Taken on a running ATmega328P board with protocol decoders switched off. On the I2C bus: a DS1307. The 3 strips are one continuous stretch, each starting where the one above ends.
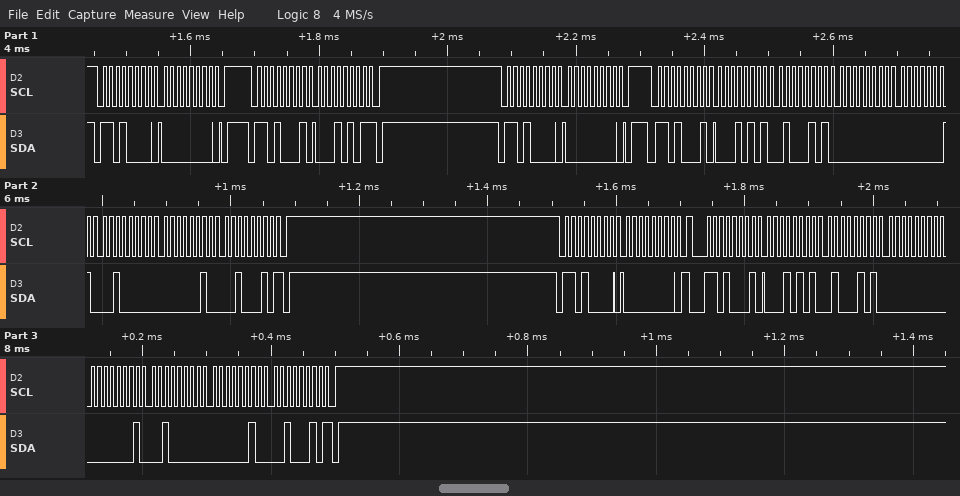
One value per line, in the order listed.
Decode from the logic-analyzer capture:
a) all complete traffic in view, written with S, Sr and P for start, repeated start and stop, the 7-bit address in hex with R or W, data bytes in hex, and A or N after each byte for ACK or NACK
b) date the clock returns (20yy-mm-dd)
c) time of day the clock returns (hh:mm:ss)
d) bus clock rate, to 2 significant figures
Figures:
S 68W A 00 A P S 68R A 15 N P S 68W A 00 A P S 68R A 15 A 45 A 00 A 01 A 20 A 02 A 22 N P S 68W A 00 A Sr 68R A 15 A 45 A 00 A 01 A 20 A 02 A 22 N P
2022-02-20
00:45:15
100 kHz
